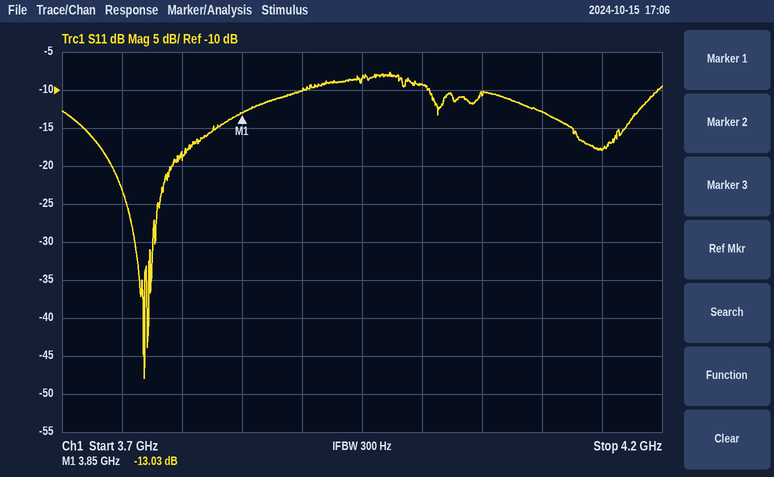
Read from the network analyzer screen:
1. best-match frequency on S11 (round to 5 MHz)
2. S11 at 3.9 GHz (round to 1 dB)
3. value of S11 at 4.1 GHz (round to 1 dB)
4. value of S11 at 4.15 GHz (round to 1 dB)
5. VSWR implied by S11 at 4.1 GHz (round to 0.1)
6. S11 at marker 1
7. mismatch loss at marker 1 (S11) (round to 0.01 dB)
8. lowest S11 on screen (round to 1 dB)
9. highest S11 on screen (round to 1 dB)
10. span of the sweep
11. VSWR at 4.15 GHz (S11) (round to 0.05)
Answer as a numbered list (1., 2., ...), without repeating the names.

1. 3.770 GHz
2. -10 dB
3. -13 dB
4. -18 dB
5. 1.6
6. -13.03 dB
7. 0.22 dB
8. -48 dB
9. -8 dB
10. 500 MHz
11. 1.30
